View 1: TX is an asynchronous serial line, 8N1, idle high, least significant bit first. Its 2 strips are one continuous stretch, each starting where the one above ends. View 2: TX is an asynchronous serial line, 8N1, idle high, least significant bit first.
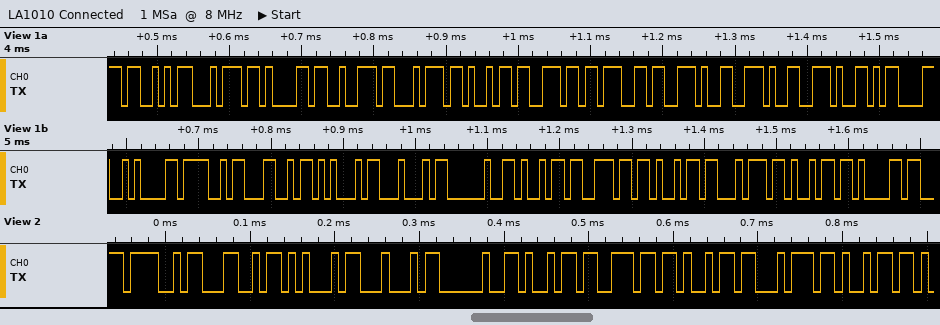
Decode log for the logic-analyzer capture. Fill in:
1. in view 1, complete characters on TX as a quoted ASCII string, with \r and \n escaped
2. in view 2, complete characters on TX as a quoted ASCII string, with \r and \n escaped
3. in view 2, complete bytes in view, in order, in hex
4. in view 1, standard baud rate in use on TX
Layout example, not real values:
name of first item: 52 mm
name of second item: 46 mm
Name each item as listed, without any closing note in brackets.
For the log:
in view 1, complete characters on TX as a quoted ASCII string, with \r and \n escaped: "Starting...\r\nOLED initia"
in view 2, complete characters on TX as a quoted ASCII string, with \r and \n escaped: "OLED initi"
in view 2, complete bytes in view, in order, in hex: 4F 4C 45 44 20 69 6E 69 74 69
in view 1, standard baud rate in use on TX: 115200 baud
